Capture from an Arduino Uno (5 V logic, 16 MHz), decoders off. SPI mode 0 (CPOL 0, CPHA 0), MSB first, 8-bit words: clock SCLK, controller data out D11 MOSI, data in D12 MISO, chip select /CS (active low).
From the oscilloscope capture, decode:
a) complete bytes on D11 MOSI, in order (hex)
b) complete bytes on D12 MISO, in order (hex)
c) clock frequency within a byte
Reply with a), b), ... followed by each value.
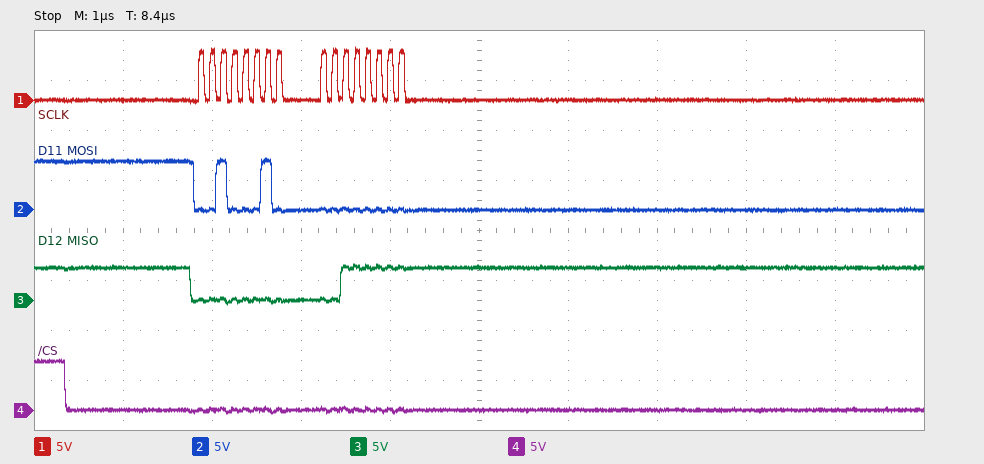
a) 22 00
b) 00 3F
c) 8 MHz
